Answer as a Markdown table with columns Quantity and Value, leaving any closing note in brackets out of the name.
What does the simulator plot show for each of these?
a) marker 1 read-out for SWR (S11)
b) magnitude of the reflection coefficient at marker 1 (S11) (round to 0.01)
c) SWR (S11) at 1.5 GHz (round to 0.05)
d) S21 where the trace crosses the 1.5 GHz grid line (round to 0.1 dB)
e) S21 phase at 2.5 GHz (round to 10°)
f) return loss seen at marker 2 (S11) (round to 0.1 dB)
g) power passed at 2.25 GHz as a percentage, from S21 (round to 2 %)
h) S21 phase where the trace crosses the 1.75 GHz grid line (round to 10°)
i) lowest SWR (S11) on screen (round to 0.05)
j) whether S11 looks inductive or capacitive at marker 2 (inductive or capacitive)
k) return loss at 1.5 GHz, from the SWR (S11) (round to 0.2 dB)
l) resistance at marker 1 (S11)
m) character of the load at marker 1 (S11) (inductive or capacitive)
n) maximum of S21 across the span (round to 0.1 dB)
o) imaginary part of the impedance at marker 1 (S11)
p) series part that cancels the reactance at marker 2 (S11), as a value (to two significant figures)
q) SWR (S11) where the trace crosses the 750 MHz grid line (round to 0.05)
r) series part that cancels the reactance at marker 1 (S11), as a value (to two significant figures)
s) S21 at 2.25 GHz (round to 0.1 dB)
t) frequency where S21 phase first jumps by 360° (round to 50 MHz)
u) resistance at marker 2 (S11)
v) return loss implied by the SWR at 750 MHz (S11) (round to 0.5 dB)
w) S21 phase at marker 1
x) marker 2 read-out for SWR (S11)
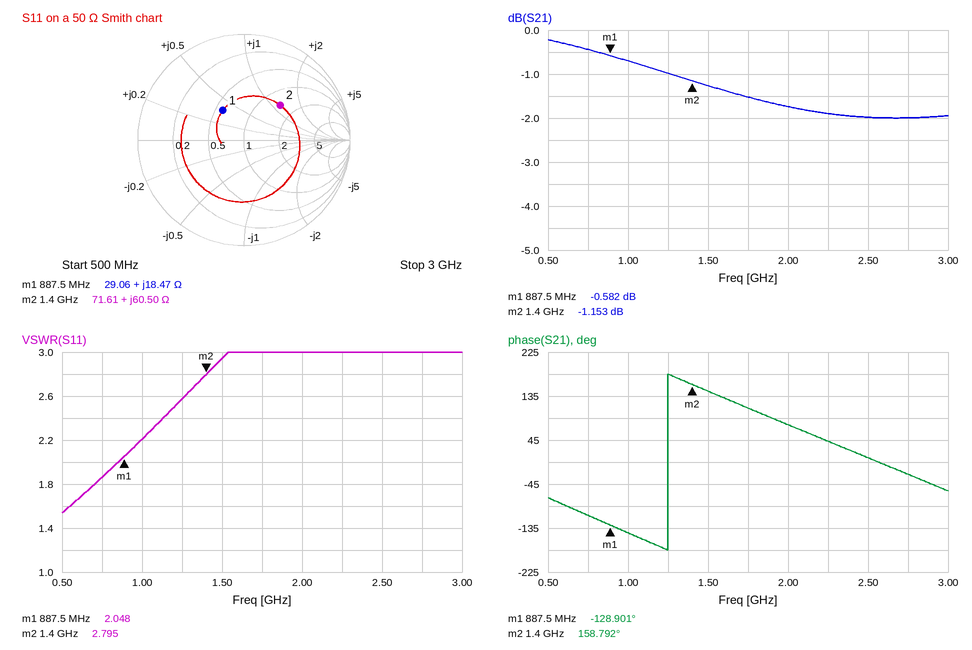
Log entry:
| Quantity | Value |
|---|---|
| marker 1 read-out for SWR | 2.048 |
| magnitude of the reflection coefficient at marker 1 (S11) | 0.34 |
| SWR (S11) at 1.5 GHz | 2.95 |
| S21 where the trace crosses the 1.5 GHz grid line | -1.3 dB |
| S21 phase at 2.5 GHz | 10° |
| return loss seen at marker 2 (S11) | 6.5 dB |
| power passed at 2.25 GHz as a percentage, from S21 | 64 % |
| S21 phase where the trace crosses the 1.75 GHz grid line | 110° |
| lowest SWR (S11) on screen | 1.55 |
| whether S11 looks inductive or capacitive at marker 2 | inductive |
| return loss at 1.5 GHz, from the SWR (S11) | 6.2 dB |
| resistance at marker 1 | 29.06 Ω |
| character of the load at marker 1 (S11) | inductive |
| maximum of S21 across the span | -0.2 dB |
| imaginary part of the impedance at marker 1 | +18.47 Ω |
| series part that cancels the reactance at marker 2 (S11), as a value | 1.9 pF |
| SWR (S11) where the trace crosses the 750 MHz grid line | 1.85 |
| series part that cancels the reactance at marker 1 (S11), as a value | 9.7 pF |
| S21 at 2.25 GHz | -1.9 dB |
| frequency where S21 phase first jumps by 360° | 1.25 GHz |
| resistance at marker 2 | 71.61 Ω |
| return loss implied by the SWR at 750 MHz (S11) | 10.5 dB |
| S21 phase at marker 1 | -128.901° |
| marker 2 read-out for SWR | 2.795 |
